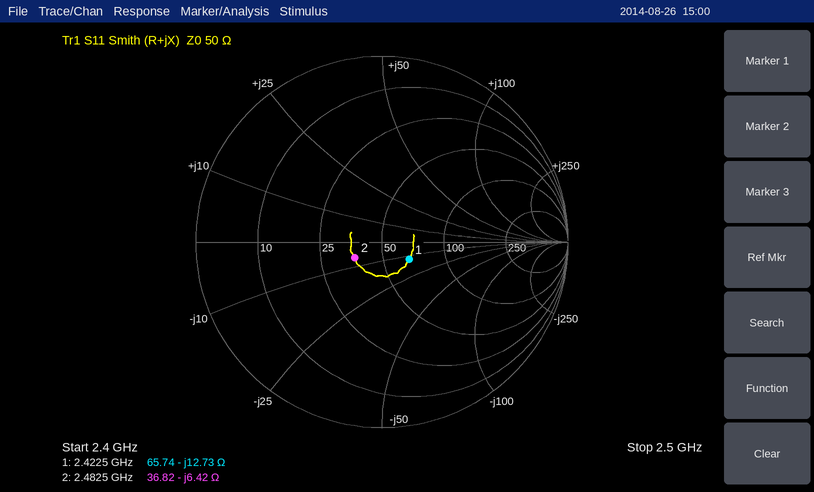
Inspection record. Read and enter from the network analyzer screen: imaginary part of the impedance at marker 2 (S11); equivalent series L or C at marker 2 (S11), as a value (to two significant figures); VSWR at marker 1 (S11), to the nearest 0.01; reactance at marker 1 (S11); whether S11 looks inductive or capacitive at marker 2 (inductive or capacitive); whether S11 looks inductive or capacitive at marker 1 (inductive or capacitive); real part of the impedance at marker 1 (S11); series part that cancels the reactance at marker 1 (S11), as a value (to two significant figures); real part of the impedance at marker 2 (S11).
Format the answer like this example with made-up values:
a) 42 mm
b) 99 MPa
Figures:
a) -6.42 Ω
b) 10.0 pF
c) 1.42
d) -12.73 Ω
e) capacitive
f) capacitive
g) 65.74 Ω
h) 840 pH
i) 36.82 Ω
